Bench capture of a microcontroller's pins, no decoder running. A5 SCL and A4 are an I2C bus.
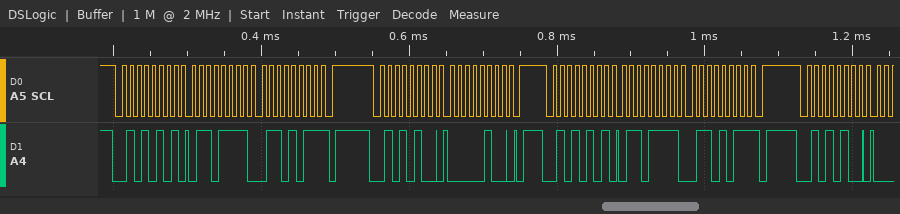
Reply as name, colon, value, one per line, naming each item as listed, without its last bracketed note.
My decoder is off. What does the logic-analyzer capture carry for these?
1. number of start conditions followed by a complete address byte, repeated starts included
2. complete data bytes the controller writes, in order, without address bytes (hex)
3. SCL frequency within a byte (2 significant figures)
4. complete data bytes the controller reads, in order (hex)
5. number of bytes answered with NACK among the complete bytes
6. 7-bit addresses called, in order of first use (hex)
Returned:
number of start conditions followed by a complete address byte, repeated starts included: 4
complete data bytes the controller writes, in order, without address bytes: 04
SCL frequency within a byte: 100 kHz
complete data bytes the controller reads, in order: 6F 6B 6F 6B
number of bytes answered with NACK among the complete bytes: 2
7-bit addresses called, in order of first use: 0x2A
